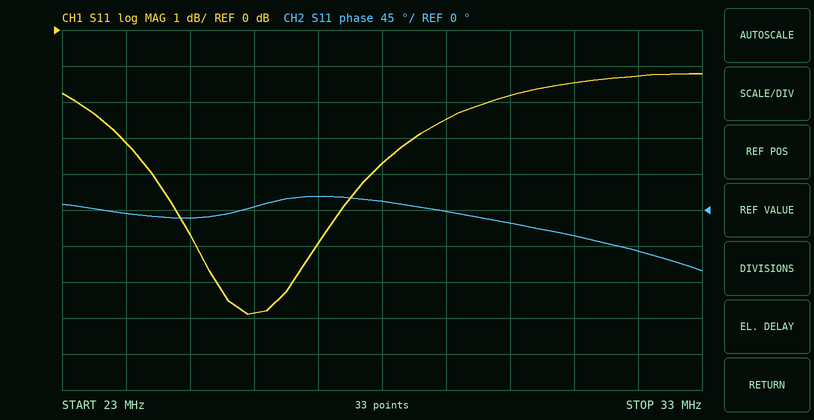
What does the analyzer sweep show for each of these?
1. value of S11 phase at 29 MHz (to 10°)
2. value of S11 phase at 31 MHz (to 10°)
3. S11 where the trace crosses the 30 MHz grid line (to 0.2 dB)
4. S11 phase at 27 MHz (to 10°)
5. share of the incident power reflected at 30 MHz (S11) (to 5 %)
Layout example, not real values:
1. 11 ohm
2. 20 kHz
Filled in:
1. 0°
2. -30°
3. -1.8 dB
4. 20°
5. 65 %
